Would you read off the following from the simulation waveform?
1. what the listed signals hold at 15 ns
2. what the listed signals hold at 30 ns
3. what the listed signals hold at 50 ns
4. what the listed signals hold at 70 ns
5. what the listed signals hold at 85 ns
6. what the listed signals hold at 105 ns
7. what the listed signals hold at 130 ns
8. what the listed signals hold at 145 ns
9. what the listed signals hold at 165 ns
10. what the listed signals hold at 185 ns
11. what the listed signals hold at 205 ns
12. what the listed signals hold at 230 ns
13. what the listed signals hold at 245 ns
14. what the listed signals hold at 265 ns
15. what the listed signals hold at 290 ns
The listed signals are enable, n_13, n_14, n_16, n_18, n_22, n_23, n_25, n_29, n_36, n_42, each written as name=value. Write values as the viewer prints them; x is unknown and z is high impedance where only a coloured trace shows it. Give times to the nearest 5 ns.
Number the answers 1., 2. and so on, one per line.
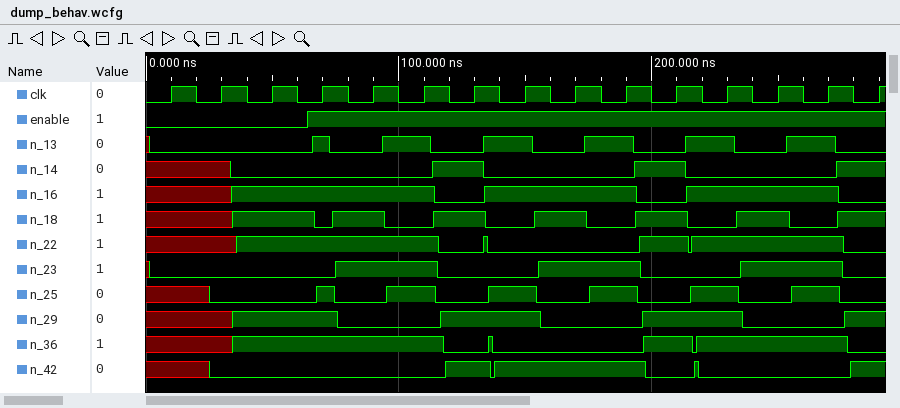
1. enable=0, n_13=0, n_14=x, n_16=x, n_18=x, n_22=x, n_23=0, n_25=x, n_29=x, n_36=x, n_42=x
2. enable=0, n_13=0, n_14=x, n_16=x, n_18=x, n_22=x, n_23=0, n_25=0, n_29=x, n_36=x, n_42=0
3. enable=0, n_13=0, n_14=0, n_16=1, n_18=1, n_22=1, n_23=0, n_25=0, n_29=1, n_36=1, n_42=0
4. enable=1, n_13=1, n_14=0, n_16=1, n_18=0, n_22=1, n_23=0, n_25=1, n_29=1, n_36=1, n_42=0
5. enable=1, n_13=0, n_14=0, n_16=1, n_18=1, n_22=1, n_23=1, n_25=0, n_29=0, n_36=1, n_42=0
6. enable=1, n_13=1, n_14=0, n_16=1, n_18=0, n_22=1, n_23=1, n_25=1, n_29=0, n_36=1, n_42=0
7. enable=1, n_13=0, n_14=1, n_16=0, n_18=1, n_22=0, n_23=0, n_25=0, n_29=1, n_36=0, n_42=1
8. enable=1, n_13=1, n_14=0, n_16=1, n_18=0, n_22=0, n_23=0, n_25=1, n_29=1, n_36=0, n_42=1
9. enable=1, n_13=0, n_14=0, n_16=1, n_18=1, n_22=0, n_23=1, n_25=0, n_29=0, n_36=0, n_42=1
10. enable=1, n_13=1, n_14=0, n_16=1, n_18=0, n_22=0, n_23=1, n_25=1, n_29=0, n_36=0, n_42=1
11. enable=1, n_13=0, n_14=1, n_16=0, n_18=1, n_22=1, n_23=0, n_25=0, n_29=1, n_36=1, n_42=0
12. enable=1, n_13=1, n_14=0, n_16=1, n_18=0, n_22=1, n_23=0, n_25=1, n_29=1, n_36=1, n_42=0
13. enable=1, n_13=0, n_14=0, n_16=1, n_18=1, n_22=1, n_23=1, n_25=0, n_29=0, n_36=1, n_42=0
14. enable=1, n_13=1, n_14=0, n_16=1, n_18=0, n_22=1, n_23=1, n_25=1, n_29=0, n_36=1, n_42=0
15. enable=1, n_13=0, n_14=1, n_16=0, n_18=1, n_22=0, n_23=0, n_25=0, n_29=1, n_36=0, n_42=1
